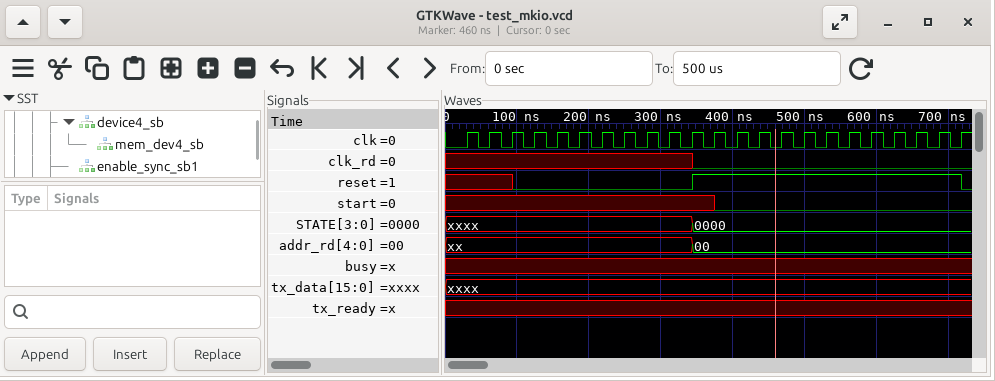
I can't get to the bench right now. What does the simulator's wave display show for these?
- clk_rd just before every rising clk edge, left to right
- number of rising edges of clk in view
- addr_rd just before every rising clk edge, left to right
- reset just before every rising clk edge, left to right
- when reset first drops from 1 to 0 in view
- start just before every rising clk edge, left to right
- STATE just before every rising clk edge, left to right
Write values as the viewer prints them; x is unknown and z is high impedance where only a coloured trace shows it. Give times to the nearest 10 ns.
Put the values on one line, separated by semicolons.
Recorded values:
x x x x x x x x x x x 0 0 0 0 0 0 0 0 0 0 0 0; 23; xx, xx, xx, xx, xx, xx, xx, xx, xx, xx, xx, 00, 00, 00, 00, 00, 00, 00, 00, 00, 00, 00, 00; x x x 0 0 0 0 0 0 0 0 1 1 1 1 1 1 1 1 1 1 1 1; 720 ns; x x x x x x x x x x x x 0 0 0 0 0 0 0 0 0 0 0; xxxx, xxxx, xxxx, xxxx, xxxx, xxxx, xxxx, xxxx, xxxx, xxxx, xxxx, 0000, 0000, 0000, 0000, 0000, 0000, 0000, 0000, 0000, 0000, 0000, 0000
